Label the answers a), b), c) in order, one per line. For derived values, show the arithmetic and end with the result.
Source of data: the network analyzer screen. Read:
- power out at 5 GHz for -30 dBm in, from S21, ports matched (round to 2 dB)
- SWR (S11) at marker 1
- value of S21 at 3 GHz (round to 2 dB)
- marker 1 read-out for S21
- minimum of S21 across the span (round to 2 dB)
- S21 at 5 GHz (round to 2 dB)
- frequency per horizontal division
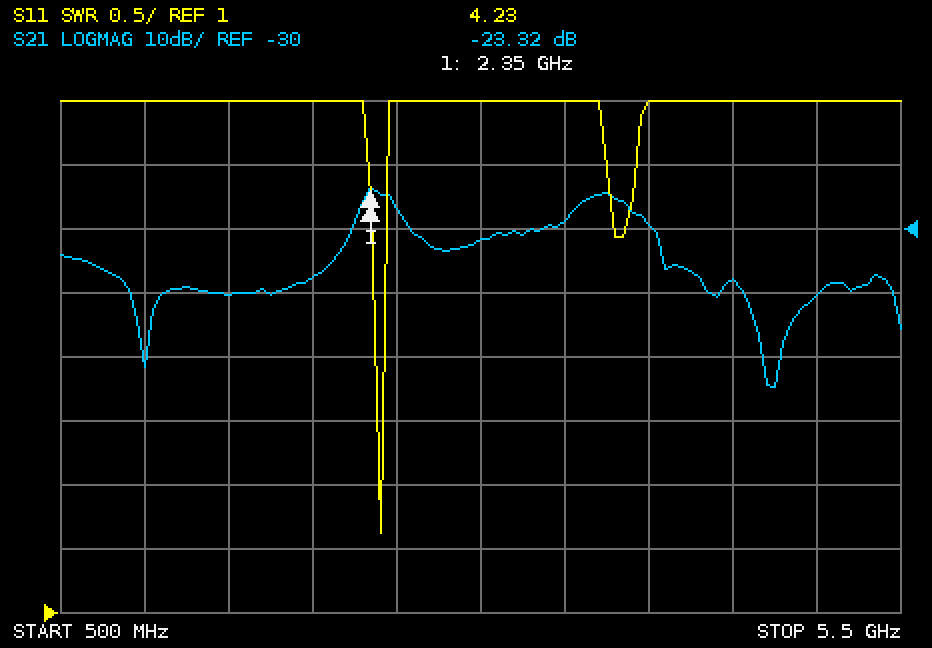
a) -30 dBm + (-40 dB) = -70 dBm
b) 4.23
c) -32 dB
d) -23.32 dB
e) -54 dB
f) -40 dB
g) 500 MHz
